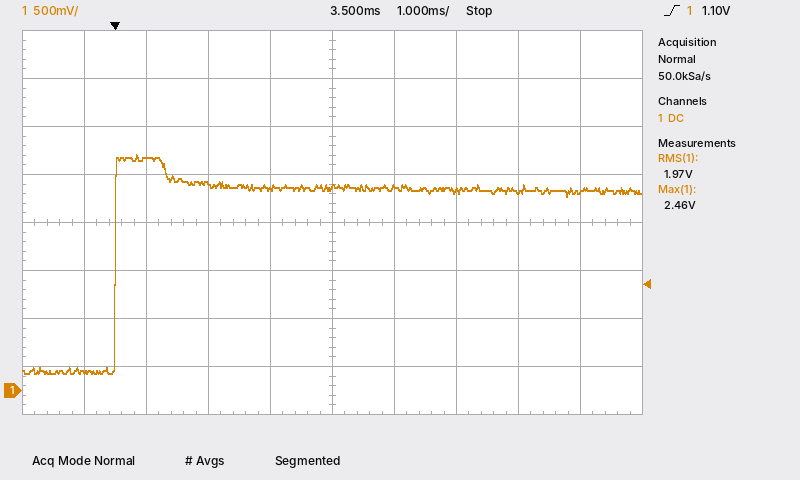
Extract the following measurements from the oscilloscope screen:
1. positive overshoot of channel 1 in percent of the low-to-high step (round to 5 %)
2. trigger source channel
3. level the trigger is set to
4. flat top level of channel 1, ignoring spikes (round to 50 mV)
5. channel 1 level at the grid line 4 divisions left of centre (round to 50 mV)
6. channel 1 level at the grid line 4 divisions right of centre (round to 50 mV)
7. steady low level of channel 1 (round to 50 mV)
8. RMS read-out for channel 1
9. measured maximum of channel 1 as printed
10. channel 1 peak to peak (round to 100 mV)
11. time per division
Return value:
20 %
channel 1
1.10 V
2.10 V
200 mV
2.05 V
200 mV
1.97 V
2.46 V
2.30 V
1 ms
